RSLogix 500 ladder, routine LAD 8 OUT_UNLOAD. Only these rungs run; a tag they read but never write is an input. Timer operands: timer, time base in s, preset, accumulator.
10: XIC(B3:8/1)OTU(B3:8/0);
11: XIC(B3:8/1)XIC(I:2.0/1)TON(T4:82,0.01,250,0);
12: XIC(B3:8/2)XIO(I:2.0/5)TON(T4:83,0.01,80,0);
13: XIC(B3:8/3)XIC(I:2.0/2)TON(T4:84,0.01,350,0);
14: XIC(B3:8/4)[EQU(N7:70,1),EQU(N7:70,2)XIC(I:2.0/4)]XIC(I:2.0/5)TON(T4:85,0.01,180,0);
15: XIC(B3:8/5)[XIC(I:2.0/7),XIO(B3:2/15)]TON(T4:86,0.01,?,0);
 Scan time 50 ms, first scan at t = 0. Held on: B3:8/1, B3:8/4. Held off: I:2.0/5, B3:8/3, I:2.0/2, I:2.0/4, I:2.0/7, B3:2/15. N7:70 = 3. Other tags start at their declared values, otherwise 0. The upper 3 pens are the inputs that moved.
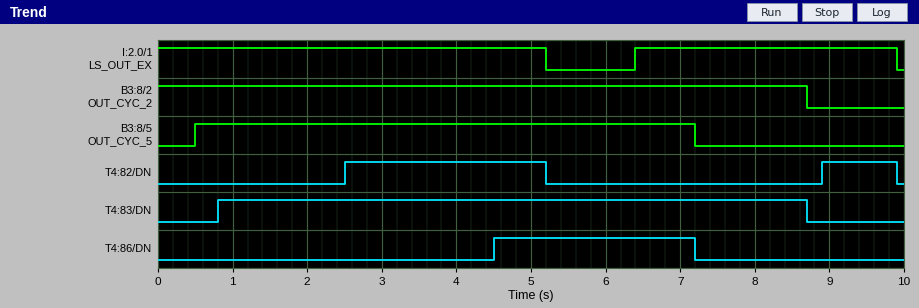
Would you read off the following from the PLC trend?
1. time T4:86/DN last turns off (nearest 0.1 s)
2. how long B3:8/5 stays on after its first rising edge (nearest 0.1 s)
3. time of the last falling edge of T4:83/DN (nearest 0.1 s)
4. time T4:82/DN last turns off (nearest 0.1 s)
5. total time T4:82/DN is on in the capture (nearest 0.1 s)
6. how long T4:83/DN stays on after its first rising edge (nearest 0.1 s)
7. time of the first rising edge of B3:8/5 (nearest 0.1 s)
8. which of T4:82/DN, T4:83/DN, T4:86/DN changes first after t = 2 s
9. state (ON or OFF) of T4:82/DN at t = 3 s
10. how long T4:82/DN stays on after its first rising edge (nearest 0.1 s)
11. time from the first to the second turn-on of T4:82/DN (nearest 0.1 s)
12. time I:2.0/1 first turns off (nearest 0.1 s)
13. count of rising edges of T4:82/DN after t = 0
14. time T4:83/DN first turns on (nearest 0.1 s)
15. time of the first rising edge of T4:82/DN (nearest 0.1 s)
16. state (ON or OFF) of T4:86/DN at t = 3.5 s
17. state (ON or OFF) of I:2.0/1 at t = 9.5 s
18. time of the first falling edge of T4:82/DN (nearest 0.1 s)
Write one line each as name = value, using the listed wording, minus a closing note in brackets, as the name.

time T4:86/DN last turns off = 7.2 s
how long B3:8/5 stays on after its first rising edge = 6.7 s
time of the last falling edge of T4:83/DN = 8.7 s
time T4:82/DN last turns off = 9.9 s
total time T4:82/DN is on in the capture = 3.7 s
how long T4:83/DN stays on after its first rising edge = 7.9 s
time of the first rising edge of B3:8/5 = 0.5 s
which of T4:82/DN, T4:83/DN, T4:86/DN changes first after t = 2 s = T4:82/DN
state (ON or OFF) of T4:82/DN at t = 3 s = ON
how long T4:82/DN stays on after its first rising edge = 2.7 s
time from the first to the second turn-on of T4:82/DN = 6.4 s
time I:2.0/1 first turns off = 5.2 s
count of rising edges of T4:82/DN after t = 0 = 2
time T4:83/DN first turns on = 0.8 s
time of the first rising edge of T4:82/DN = 2.5 s
state (ON or OFF) of T4:86/DN at t = 3.5 s = OFF
state (ON or OFF) of I:2.0/1 at t = 9.5 s = ON
time of the first falling edge of T4:82/DN = 5.2 s
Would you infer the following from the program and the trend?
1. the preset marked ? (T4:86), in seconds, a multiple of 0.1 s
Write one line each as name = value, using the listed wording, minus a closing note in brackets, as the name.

the preset marked ? (T4:86), in seconds, a multiple of 0.1 s = 4.0 s
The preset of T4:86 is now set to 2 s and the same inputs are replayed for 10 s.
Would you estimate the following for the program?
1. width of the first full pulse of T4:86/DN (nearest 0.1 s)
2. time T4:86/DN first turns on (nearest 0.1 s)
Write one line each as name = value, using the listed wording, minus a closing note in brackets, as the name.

width of the first full pulse of T4:86/DN = 4.7 s
time T4:86/DN first turns on = 2.5 s
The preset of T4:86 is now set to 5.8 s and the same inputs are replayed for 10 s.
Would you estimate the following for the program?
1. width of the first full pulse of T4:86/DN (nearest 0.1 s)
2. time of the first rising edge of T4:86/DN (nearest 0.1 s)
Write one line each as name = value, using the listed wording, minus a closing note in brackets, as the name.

width of the first full pulse of T4:86/DN = 0.9 s
time of the first rising edge of T4:86/DN = 6.3 s
